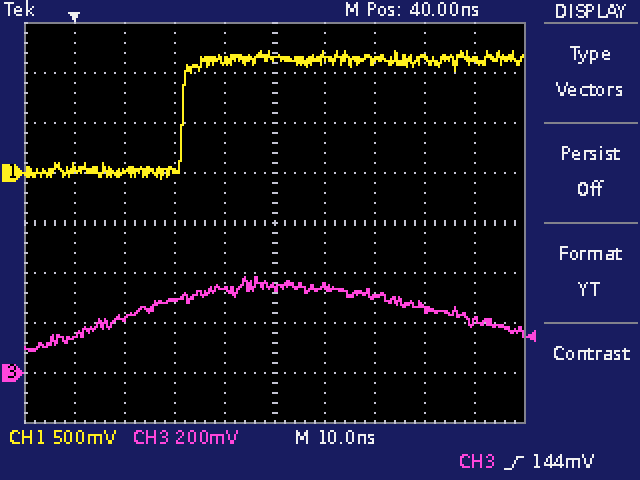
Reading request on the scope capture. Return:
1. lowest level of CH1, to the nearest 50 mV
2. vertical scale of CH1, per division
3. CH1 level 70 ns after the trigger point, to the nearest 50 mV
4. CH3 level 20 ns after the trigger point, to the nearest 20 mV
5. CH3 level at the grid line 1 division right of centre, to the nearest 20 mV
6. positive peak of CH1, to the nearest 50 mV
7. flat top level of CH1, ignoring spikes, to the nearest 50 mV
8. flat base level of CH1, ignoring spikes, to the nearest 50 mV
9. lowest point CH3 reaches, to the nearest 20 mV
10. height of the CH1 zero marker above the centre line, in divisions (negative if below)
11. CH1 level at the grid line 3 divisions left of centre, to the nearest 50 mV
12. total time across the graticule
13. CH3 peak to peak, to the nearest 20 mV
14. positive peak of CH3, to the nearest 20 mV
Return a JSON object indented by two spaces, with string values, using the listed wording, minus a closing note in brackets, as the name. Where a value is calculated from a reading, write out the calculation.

{
  "lowest level of CH1, to the nearest 50 mV": "-50 mV",
  "vertical scale of CH1, per division": "500 mV",
  "CH1 level 70 ns after the trigger point, to the nearest 50 mV": "1.15 V",
  "CH3 level 20 ns after the trigger point, to the nearest 20 mV": "300 mV",
  "CH3 level at the grid line 1 division right of centre, to the nearest 20 mV": "340 mV",
  "positive peak of CH1, to the nearest 50 mV": "1.20 V",
  "flat top level of CH1, ignoring spikes, to the nearest 50 mV": "1.15 V",
  "flat base level of CH1, ignoring spikes, to the nearest 50 mV": "0 mV",
  "lowest point CH3 reaches, to the nearest 20 mV": "80 mV",
  "height of the CH1 zero marker above the centre line, in divisions": "+1.0 div",
  "CH1 level at the grid line 3 divisions left of centre, to the nearest 50 mV": "0 mV",
  "total time across the graticule": "100 ns",
  "CH3 peak to peak, to the nearest 20 mV": "380 mV − (80 mV) = 300 mV",
  "positive peak of CH3, to the nearest 20 mV": "380 mV"
}
